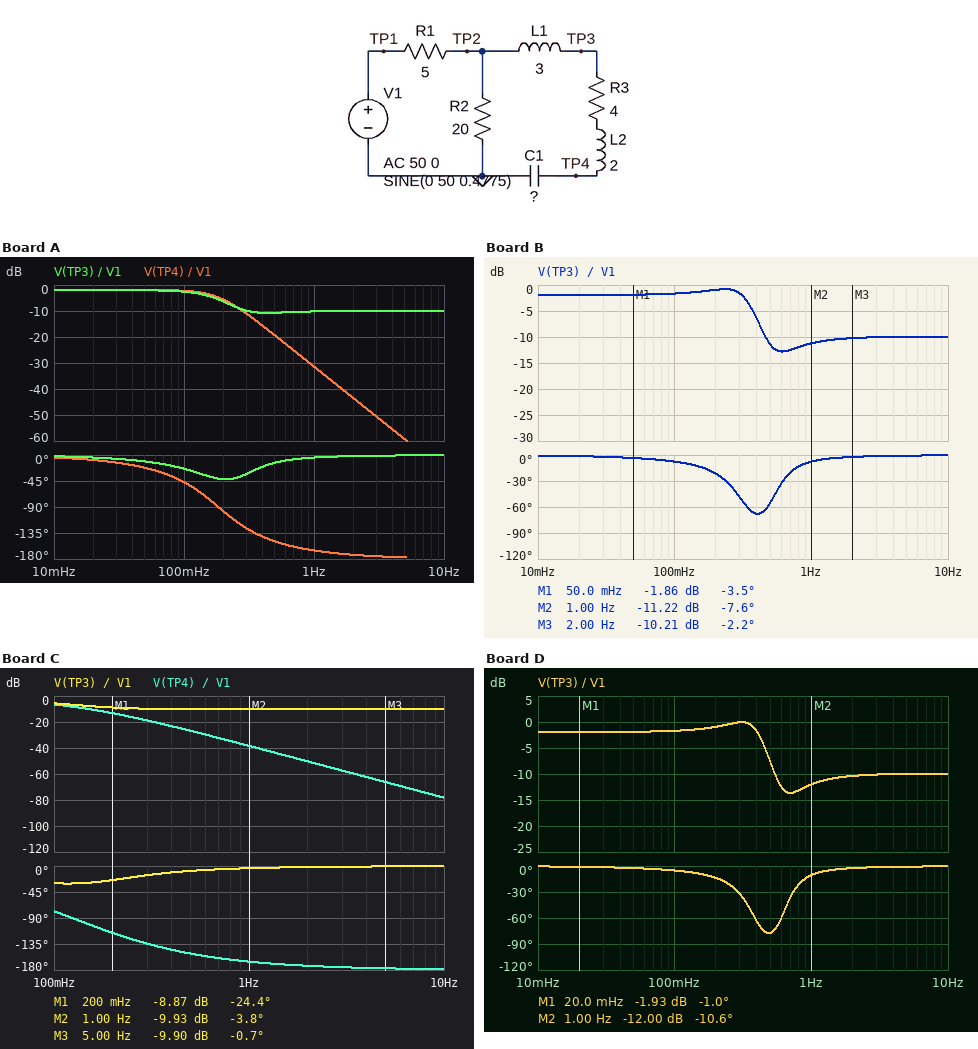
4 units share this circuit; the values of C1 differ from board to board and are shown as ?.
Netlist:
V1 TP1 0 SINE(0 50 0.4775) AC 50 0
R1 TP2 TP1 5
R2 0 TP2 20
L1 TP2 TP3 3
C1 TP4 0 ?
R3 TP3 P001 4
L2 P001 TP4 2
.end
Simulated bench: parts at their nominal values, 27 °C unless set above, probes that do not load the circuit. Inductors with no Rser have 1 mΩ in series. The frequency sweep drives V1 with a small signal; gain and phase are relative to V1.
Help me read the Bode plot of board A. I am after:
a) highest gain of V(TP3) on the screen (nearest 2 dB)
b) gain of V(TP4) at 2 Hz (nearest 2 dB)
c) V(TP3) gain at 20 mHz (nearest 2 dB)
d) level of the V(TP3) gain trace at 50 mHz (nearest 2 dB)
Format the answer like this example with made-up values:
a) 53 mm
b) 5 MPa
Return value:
a) -2 dB
b) -44 dB
c) -2 dB
d) -2 dB
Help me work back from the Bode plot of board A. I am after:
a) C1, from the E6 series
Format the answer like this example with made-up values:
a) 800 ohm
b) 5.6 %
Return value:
a) 150 mF
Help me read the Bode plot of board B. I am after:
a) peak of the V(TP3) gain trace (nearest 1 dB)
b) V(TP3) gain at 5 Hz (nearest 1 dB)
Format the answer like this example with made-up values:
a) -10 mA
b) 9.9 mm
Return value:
a) -1 dB
b) -10 dB
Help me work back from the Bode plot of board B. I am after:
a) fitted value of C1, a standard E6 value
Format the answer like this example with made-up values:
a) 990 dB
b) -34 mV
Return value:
a) 47 mF
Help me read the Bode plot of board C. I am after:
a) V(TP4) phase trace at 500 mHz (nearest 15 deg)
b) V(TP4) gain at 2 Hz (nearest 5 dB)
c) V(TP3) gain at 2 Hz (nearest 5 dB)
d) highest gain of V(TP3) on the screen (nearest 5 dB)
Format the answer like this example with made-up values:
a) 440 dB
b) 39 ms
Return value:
a) -150 deg
b) -50 dB
c) -10 dB
d) -5 dB
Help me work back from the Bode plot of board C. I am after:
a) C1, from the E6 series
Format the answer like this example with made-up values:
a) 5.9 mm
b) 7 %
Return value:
a) 330 mF
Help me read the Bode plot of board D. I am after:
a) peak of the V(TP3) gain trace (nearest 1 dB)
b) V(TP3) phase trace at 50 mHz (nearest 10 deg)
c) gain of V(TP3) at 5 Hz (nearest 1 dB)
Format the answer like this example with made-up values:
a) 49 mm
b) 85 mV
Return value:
a) 0 dB
b) 0 deg
c) -10 dB
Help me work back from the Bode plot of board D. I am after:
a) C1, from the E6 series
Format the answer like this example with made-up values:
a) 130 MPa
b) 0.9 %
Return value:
a) 33 mF
